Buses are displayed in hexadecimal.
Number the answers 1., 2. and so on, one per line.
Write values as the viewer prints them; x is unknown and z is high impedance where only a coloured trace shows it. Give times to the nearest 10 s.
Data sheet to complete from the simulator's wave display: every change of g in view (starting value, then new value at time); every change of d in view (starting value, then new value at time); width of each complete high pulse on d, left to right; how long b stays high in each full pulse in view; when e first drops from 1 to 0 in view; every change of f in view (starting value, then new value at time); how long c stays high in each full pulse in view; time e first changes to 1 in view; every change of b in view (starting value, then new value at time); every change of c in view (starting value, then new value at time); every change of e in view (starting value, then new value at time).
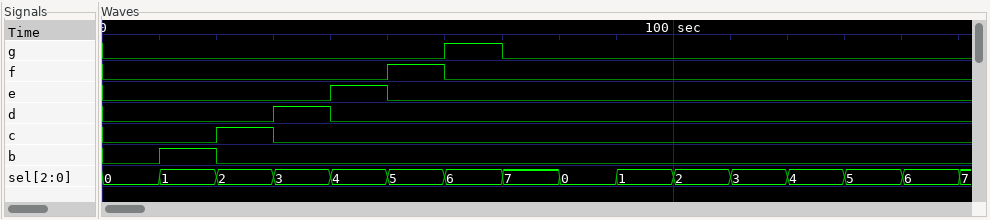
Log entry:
1. 0, 1 at 60 s, 0 at 70 s
2. 0, 1 at 30 s, 0 at 40 s
3. 10 s
4. 10 s
5. 50 s
6. 0, 1 at 50 s, 0 at 60 s
7. 10 s
8. 40 s
9. 0, 1 at 10 s, 0 at 20 s
10. 0, 1 at 20 s, 0 at 30 s
11. 0, 1 at 40 s, 0 at 50 s
